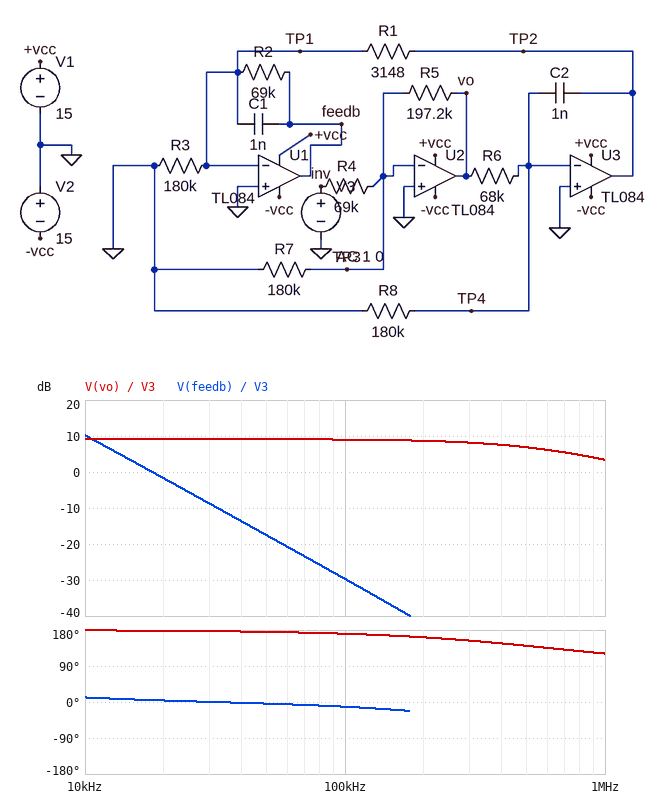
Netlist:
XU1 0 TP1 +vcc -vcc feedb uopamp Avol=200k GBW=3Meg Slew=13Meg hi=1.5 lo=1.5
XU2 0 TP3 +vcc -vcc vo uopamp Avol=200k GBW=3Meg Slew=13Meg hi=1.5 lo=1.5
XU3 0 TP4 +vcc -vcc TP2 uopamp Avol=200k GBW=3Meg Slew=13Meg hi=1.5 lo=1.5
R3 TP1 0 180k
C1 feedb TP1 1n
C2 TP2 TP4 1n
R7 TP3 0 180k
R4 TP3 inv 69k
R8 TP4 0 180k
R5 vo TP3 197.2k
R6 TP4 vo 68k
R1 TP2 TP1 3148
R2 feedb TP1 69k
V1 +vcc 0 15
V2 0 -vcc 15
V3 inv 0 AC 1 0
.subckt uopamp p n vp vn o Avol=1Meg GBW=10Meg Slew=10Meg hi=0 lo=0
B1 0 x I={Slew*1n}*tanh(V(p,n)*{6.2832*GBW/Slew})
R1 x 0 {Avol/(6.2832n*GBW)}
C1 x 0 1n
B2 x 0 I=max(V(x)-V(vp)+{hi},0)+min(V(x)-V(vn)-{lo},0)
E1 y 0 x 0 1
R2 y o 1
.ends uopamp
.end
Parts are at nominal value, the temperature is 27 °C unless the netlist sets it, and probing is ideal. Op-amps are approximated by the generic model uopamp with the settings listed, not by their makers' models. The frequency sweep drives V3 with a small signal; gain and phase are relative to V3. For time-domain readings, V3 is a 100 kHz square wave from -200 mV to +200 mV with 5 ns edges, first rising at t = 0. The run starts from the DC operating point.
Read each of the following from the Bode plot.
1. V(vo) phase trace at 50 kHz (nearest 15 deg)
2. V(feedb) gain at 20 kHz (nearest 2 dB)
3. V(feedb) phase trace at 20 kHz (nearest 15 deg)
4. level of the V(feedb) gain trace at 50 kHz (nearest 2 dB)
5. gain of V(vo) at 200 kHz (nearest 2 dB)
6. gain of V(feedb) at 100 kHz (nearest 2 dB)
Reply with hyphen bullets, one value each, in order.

- 180 deg
- -2 dB
- 0 deg
- -18 dB
- 8 dB
- -30 dB
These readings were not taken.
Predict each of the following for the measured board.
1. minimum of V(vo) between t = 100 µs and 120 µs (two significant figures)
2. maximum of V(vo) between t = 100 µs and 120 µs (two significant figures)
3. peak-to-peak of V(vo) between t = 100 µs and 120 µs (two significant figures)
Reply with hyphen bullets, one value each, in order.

- -570 mV
- 570 mV
- 1.1 V
